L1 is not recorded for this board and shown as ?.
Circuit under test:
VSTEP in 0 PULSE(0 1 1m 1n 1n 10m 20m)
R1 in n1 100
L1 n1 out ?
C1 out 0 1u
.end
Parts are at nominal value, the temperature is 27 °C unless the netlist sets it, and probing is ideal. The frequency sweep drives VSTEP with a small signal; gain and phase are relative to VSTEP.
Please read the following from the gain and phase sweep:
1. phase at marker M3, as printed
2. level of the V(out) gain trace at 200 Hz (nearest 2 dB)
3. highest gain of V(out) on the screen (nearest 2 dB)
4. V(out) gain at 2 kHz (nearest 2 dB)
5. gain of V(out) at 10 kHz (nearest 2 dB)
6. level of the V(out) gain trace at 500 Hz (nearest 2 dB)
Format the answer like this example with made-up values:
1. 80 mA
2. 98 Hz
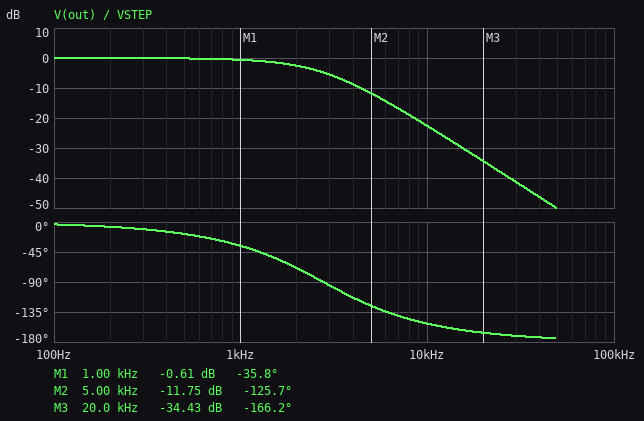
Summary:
1. -166.2 deg
2. 0 dB
3. 0 dB
4. -2 dB
5. -22 dB
6. 0 dB
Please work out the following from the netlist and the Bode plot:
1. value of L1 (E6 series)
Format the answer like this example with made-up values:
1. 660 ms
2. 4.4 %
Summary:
1. 3.3 mH
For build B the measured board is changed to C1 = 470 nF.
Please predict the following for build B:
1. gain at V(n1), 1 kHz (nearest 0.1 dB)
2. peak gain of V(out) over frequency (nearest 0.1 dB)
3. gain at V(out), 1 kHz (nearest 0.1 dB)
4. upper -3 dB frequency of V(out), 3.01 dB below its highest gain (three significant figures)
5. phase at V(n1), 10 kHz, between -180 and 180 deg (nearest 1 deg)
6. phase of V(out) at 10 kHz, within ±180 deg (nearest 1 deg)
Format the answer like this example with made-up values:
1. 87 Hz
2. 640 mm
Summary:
1. -0.4 dB
2. 0.4 dB
3. 0.1 dB
4. 4.51 kHz
5. 30 deg
6. -150 deg
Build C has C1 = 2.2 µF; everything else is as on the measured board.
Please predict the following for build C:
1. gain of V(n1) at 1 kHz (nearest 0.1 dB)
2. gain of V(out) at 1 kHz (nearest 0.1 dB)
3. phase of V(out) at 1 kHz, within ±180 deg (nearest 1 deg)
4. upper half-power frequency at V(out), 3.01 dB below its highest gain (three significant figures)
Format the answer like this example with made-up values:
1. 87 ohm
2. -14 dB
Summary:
1. -6.8 dB
2. -3.8 dB
3. -63 deg
4. 846 Hz
